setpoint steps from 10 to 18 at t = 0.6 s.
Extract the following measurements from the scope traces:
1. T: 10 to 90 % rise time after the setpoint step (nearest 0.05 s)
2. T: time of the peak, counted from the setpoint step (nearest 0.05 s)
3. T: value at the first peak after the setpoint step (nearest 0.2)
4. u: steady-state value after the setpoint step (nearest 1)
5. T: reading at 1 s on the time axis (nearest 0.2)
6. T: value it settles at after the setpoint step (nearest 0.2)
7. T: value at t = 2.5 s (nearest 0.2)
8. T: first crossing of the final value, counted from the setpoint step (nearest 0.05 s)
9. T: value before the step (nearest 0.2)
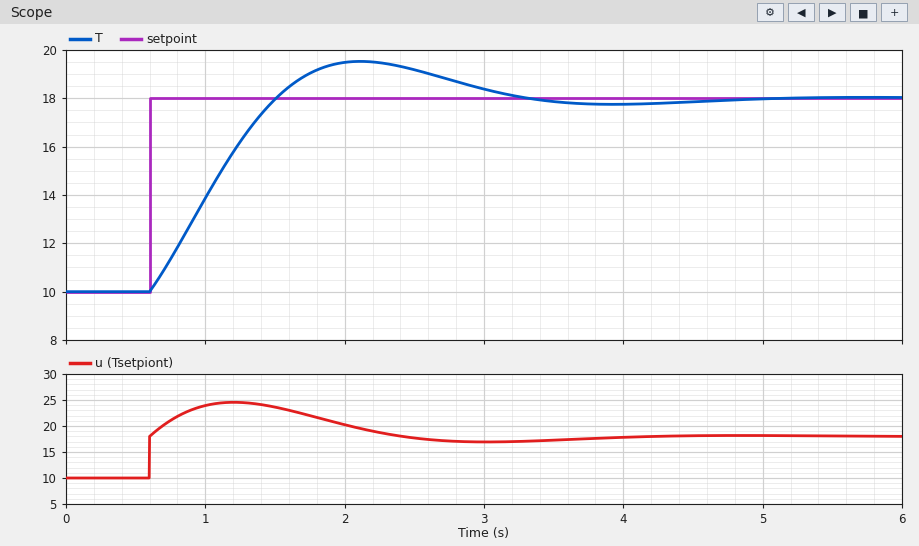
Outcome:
0.70 s
1.50 s
19.6
18
13.8
18.0
19.2
0.90 s
10.0
